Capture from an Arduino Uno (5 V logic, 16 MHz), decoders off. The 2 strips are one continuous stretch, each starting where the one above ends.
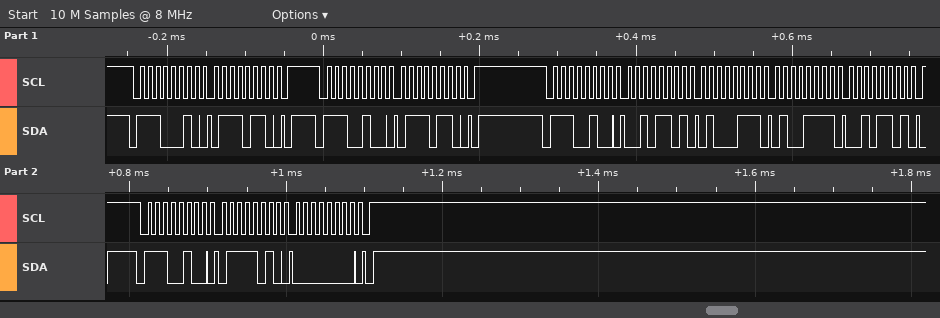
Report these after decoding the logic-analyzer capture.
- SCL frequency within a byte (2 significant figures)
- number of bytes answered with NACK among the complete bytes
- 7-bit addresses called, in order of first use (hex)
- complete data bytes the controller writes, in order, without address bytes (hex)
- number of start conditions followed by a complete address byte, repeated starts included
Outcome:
100 kHz
0
0x71 0x72
76 76 2D 47 4F 2D 7A 00
4
